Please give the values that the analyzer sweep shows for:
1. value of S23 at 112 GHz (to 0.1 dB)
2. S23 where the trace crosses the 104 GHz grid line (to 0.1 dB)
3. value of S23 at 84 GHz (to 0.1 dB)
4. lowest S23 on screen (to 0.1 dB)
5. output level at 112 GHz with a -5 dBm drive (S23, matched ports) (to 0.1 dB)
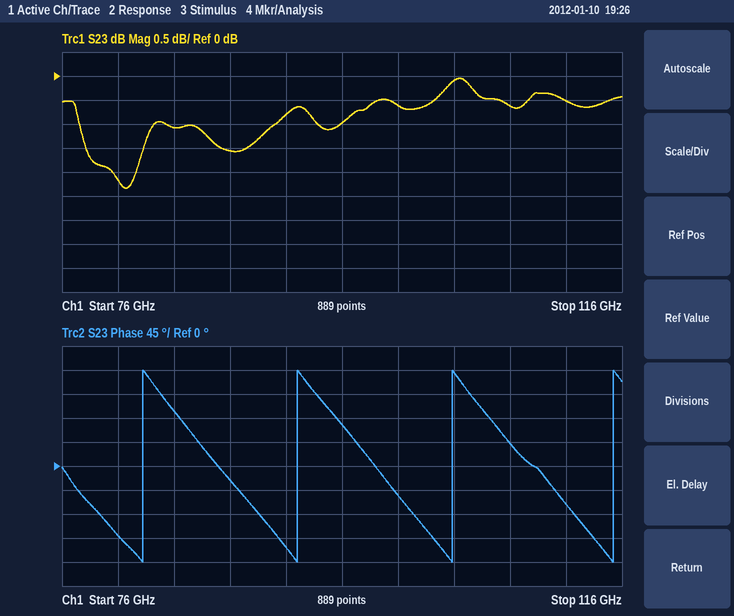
-0.5 dB
-0.1 dB
-1.1 dB
-2.3 dB
-5.5 dBm
